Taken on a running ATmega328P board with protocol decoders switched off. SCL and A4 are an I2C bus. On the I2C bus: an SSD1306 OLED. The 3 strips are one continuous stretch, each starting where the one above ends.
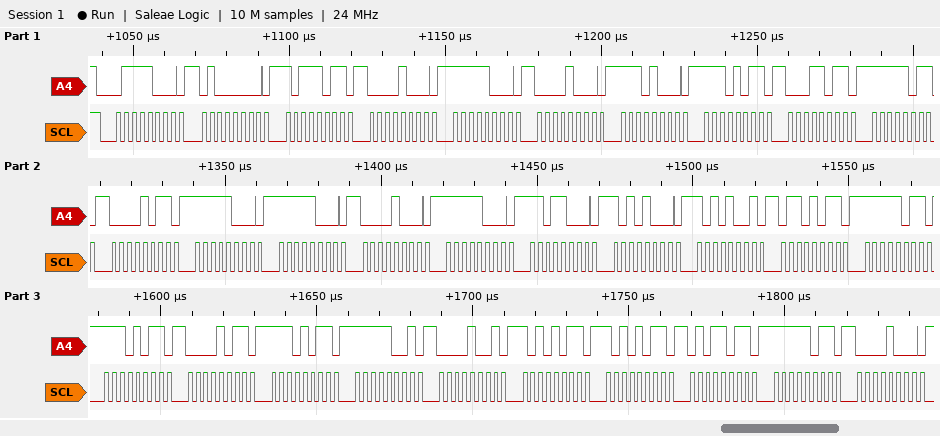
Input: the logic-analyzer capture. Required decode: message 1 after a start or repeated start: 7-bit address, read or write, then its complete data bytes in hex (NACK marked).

0x3C write: 40 BB 08 F8 08 E8 EB 1B FB 0B F8 F8 08 F8 D8 A8 A9 6B FB EB 0B EB F9 09 AB AB 5B FB 08
